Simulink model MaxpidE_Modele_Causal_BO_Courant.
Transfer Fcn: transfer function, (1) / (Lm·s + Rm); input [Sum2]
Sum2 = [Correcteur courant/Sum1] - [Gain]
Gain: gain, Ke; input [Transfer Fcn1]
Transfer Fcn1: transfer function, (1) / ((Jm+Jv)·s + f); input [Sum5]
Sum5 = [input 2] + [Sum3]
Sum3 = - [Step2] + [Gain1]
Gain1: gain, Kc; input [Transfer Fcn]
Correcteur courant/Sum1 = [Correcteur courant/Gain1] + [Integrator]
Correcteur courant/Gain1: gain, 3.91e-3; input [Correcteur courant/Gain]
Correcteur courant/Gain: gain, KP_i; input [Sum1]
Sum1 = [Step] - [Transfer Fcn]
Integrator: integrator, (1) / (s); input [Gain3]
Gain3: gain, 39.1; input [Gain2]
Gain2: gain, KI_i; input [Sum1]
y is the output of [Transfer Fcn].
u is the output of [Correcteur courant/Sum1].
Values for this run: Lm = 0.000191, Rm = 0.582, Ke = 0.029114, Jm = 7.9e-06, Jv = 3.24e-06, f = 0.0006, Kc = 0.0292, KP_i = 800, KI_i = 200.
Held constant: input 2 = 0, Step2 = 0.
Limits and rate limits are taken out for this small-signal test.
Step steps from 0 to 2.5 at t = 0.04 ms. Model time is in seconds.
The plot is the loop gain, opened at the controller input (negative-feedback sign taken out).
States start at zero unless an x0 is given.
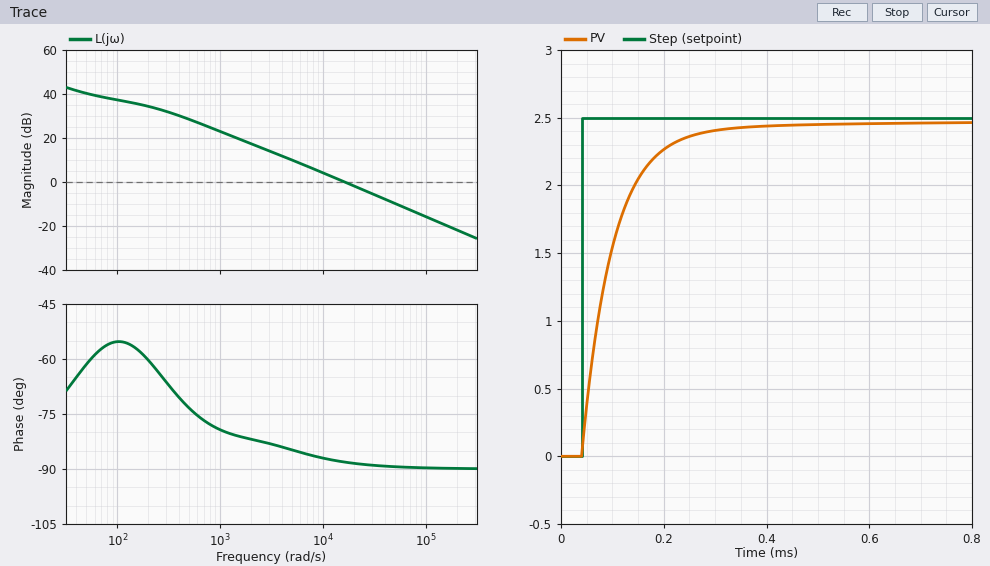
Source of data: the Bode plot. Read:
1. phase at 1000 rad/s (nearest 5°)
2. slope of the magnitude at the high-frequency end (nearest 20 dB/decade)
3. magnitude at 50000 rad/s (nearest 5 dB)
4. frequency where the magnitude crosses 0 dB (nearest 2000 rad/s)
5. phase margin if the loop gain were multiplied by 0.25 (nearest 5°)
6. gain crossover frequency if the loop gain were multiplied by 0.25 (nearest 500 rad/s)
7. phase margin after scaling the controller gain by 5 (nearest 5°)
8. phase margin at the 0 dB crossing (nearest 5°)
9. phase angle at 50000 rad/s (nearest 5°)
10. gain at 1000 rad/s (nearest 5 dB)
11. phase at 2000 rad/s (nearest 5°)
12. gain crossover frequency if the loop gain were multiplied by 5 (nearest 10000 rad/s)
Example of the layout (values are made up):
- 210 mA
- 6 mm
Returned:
- -80°
- -20 dB/decade
- -10 dB
- 16000 rad/s
- 95°
- 4000 rad/s
- 90°
- 90°
- -90°
- 25 dB
- -80°
- 80000 rad/s
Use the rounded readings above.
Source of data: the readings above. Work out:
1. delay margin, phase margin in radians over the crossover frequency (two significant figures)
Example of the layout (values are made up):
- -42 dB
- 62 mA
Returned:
- 0.000098 s
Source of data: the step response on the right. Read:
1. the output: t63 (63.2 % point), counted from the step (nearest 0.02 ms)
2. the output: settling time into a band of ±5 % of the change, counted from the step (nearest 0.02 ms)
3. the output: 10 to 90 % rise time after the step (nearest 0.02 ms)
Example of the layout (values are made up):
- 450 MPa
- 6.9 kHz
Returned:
- 0.06 ms
- 0.20 ms
- 0.14 ms
